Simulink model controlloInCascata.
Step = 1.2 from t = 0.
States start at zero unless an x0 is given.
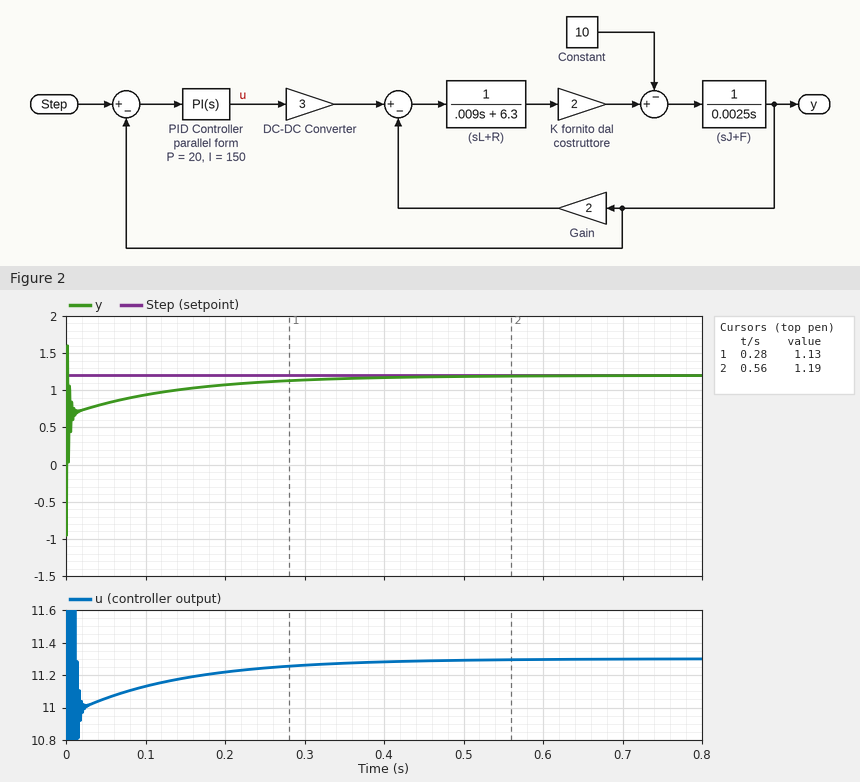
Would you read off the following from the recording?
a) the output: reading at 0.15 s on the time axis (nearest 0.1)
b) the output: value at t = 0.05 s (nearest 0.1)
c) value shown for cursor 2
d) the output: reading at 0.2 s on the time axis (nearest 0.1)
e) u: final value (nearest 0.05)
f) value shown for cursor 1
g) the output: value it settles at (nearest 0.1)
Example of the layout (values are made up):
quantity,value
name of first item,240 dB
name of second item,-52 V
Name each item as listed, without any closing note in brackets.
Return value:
quantity,value
the output: reading at 0.15 s on the time axis,1.0
the output: value at t = 0.05 s,0.8
value shown for cursor 2,1.19
the output: reading at 0.2 s on the time axis,1.1
u: final value,11.30
value shown for cursor 1,1.13
the output: value it settles at,1.2
